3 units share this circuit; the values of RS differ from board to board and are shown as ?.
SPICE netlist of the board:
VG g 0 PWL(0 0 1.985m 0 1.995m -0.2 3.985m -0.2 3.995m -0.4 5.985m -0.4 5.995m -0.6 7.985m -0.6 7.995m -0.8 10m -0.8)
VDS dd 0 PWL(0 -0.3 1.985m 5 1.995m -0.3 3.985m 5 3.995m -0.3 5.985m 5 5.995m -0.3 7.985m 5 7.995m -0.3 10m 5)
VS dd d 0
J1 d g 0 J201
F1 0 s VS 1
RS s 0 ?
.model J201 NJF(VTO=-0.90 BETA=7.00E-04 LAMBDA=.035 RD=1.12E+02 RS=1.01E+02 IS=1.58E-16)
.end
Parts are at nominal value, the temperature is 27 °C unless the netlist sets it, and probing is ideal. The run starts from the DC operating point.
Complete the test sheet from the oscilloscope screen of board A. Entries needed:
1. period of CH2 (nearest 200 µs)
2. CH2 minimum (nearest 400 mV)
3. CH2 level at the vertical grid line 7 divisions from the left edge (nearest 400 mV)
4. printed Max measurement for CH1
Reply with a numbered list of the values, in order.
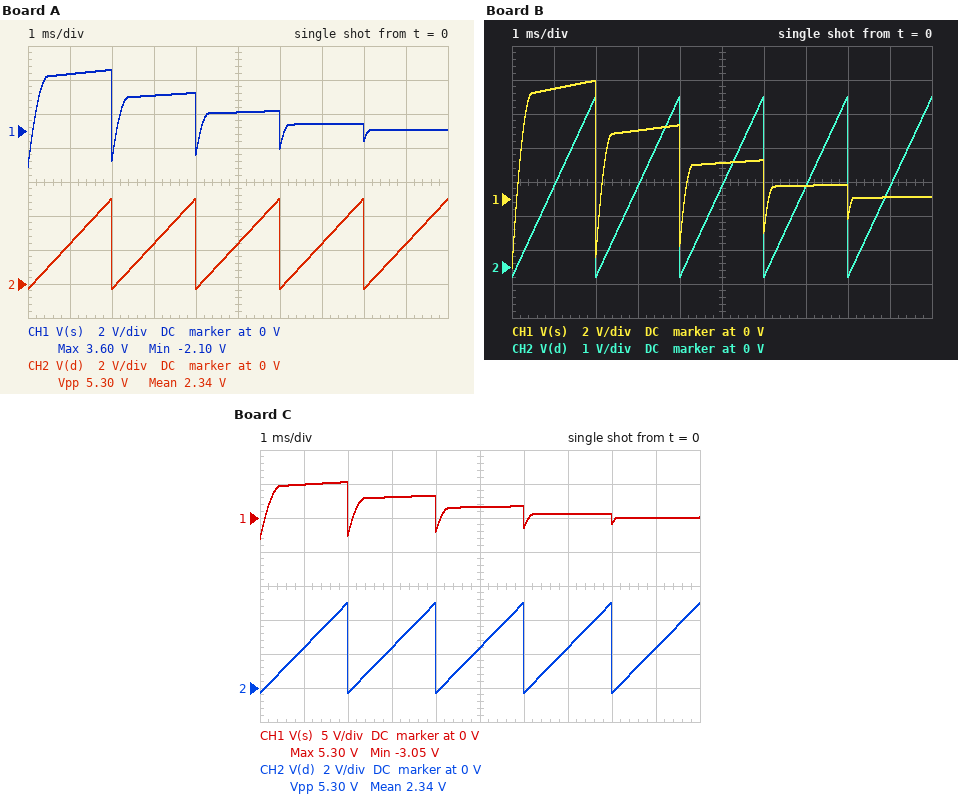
1. 2.0 ms
2. -400 mV
3. 2.4 V
4. 3.60 V
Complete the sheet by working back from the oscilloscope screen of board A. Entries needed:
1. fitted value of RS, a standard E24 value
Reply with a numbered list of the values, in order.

1. 6.2 kΩ
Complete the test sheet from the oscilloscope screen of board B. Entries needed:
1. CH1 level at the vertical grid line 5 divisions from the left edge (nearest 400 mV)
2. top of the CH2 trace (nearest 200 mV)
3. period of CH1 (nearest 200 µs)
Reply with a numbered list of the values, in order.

1. 2.0 V
2. 5.0 V
3. 2.0 ms
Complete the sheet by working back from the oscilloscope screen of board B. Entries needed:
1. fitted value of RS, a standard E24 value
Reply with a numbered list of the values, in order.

1. 12 kΩ
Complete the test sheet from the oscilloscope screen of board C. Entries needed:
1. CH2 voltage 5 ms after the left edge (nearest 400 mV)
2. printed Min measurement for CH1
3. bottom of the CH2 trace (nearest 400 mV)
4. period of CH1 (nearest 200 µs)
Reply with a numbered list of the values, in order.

1. 2.4 V
2. -3.05 V
3. -400 mV
4. 2.0 ms
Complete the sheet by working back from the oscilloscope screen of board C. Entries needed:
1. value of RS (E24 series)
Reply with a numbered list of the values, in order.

1. 9.1 kΩ
